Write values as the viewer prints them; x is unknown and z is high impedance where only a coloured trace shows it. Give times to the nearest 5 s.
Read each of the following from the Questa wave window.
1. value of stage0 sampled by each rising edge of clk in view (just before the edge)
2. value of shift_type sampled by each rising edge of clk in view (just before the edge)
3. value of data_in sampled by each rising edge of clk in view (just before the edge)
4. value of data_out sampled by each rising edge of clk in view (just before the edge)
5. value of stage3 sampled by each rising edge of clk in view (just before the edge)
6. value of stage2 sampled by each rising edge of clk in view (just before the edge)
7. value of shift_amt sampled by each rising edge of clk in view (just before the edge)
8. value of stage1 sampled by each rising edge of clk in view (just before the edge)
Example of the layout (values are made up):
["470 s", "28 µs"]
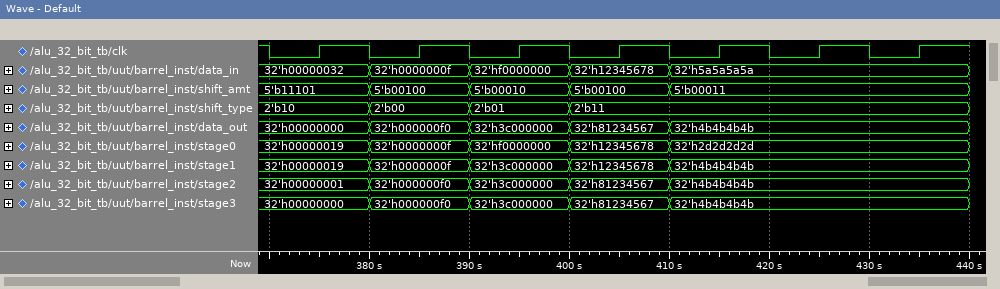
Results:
["32'h00000019, 32'h0000000f, 32'hf0000000, 32'h12345678, 32'h2d2d2d2d, 32'h2d2d2d2d, 32'h2d2d2d2d", "2'b10, 2'b00, 2'b01, 2'b11, 2'b11, 2'b11, 2'b11", "32'h00000032, 32'h0000000f, 32'hf0000000, 32'h12345678, 32'h5a5a5a5a, 32'h5a5a5a5a, 32'h5a5a5a5a", "32'h00000000, 32'h000000f0, 32'h3c000000, 32'h81234567, 32'h4b4b4b4b, 32'h4b4b4b4b, 32'h4b4b4b4b", "32'h00000000, 32'h000000f0, 32'h3c000000, 32'h81234567, 32'h4b4b4b4b, 32'h4b4b4b4b, 32'h4b4b4b4b", "32'h00000001, 32'h000000f0, 32'h3c000000, 32'h81234567, 32'h4b4b4b4b, 32'h4b4b4b4b, 32'h4b4b4b4b", "5'b11101, 5'b00100, 5'b00010, 5'b00100, 5'b00011, 5'b00011, 5'b00011", "32'h00000019, 32'h0000000f, 32'h3c000000, 32'h12345678, 32'h4b4b4b4b, 32'h4b4b4b4b, 32'h4b4b4b4b"]
